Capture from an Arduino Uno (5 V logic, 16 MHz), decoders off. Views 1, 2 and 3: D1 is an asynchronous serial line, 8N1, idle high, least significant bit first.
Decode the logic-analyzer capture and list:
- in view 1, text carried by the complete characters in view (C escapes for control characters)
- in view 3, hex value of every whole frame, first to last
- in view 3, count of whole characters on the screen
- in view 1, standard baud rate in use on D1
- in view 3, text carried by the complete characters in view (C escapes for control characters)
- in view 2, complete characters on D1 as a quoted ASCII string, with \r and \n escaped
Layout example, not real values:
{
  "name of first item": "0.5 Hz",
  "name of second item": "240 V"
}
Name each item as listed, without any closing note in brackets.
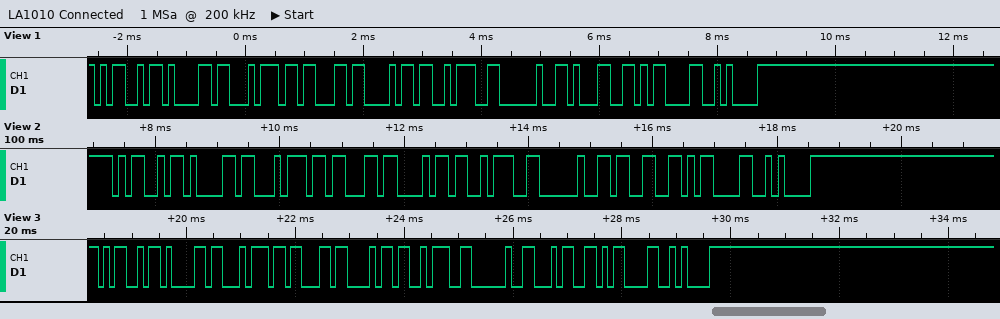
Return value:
{
  "in view 1, text carried by the complete characters in view": "\"Match: 1\\r\\n\"",
  "in view 3, hex value of every whole frame, first to last": "4D 61 74 63 68 3A 20 34 0D 0A",
  "in view 3, count of whole characters on the screen": "10",
  "in view 1, standard baud rate in use on D1": "9600 baud",
  "in view 3, text carried by the complete characters in view": "\"Match: 4\\r\\n\"",
  "in view 2, complete characters on D1 as a quoted ASCII string, with \\r and \\n escaped": "\"Match: 3\\r\\n\""
}
